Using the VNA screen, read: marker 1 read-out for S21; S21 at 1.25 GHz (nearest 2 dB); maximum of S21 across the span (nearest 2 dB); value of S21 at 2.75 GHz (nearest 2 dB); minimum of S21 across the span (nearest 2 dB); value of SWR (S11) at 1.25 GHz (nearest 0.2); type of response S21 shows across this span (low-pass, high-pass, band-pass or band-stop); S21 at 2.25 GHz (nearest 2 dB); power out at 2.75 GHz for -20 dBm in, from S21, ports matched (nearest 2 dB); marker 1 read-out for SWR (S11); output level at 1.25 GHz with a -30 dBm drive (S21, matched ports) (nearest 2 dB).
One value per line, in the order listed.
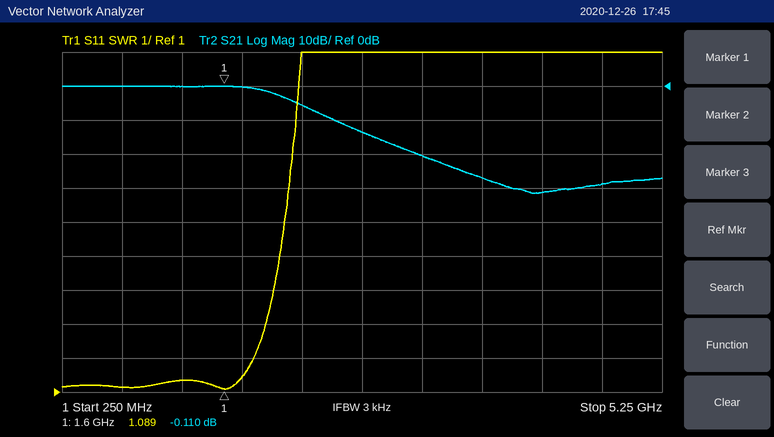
-0.110 dB
0 dB
0 dB
-14 dB
-32 dB
1.4
low-pass
-6 dB
-34 dBm
1.089
-30 dBm
